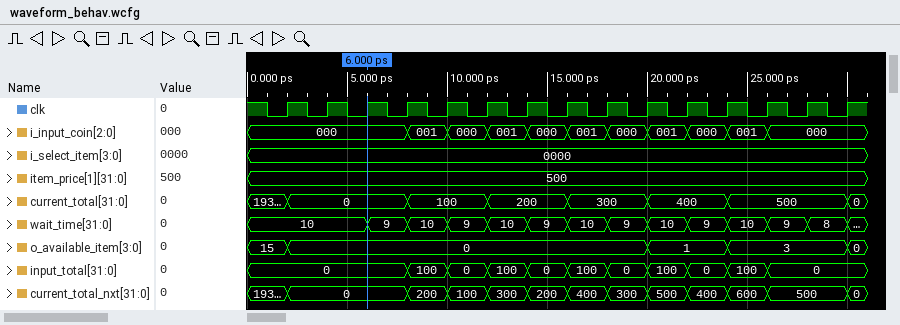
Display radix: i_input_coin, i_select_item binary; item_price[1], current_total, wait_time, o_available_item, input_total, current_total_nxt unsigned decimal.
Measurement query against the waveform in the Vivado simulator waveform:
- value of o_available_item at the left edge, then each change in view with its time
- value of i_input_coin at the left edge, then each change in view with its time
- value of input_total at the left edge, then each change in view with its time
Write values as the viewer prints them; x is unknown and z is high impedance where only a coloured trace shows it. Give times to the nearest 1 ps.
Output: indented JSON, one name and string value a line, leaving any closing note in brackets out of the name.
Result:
{
  "value of o_available_item at the left edge, then each change in view with its time": "15, 0 at 2 ps, 1 at 20 ps, 3 at 24 ps, 0 at 30 ps",
  "value of i_input_coin at the left edge, then each change in view with its time": "000, 001 at 8 ps, 000 at 10 ps, 001 at 12 ps, 000 at 14 ps, 001 at 16 ps, 000 at 18 ps, 001 at 20 ps, 000 at 22 ps, 001 at 24 ps, 000 at 26 ps",
  "value of input_total at the left edge, then each change in view with its time": "0, 100 at 8 ps, 0 at 10 ps, 100 at 12 ps, 0 at 14 ps, 100 at 16 ps, 0 at 18 ps, 100 at 20 ps, 0 at 22 ps, 100 at 24 ps, 0 at 26 ps"
}
